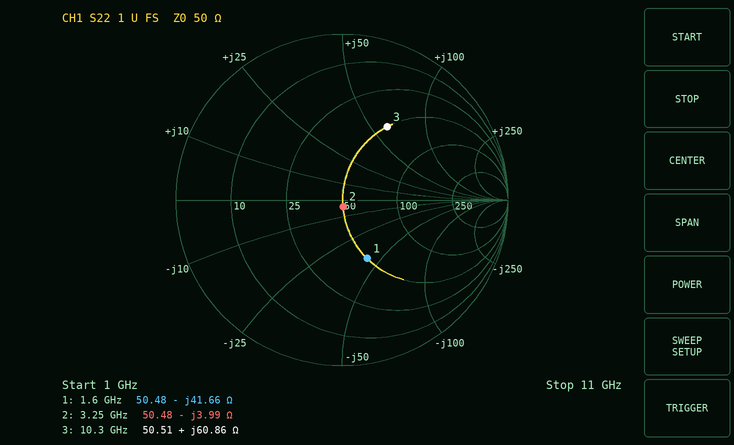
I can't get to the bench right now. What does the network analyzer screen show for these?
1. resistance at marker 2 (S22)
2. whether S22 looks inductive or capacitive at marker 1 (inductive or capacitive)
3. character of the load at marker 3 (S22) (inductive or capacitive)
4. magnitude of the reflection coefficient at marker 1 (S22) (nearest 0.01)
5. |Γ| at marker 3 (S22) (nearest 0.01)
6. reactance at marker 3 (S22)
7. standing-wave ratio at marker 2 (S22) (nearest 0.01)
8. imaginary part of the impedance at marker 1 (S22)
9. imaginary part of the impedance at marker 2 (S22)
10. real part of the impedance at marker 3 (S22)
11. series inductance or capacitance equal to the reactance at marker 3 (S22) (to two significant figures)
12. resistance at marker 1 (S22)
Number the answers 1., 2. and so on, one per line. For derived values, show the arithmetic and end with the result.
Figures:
1. 50.48 Ω
2. capacitive
3. inductive
4. 0.38
5. 0.52
6. +60.86 Ω
7. 1.08
8. -41.66 Ω
9. -3.99 Ω
10. 50.51 Ω
11. L = 60.86 Ω/(2π × 10.3 GHz) ≈ 940 pH
12. 50.48 Ω
